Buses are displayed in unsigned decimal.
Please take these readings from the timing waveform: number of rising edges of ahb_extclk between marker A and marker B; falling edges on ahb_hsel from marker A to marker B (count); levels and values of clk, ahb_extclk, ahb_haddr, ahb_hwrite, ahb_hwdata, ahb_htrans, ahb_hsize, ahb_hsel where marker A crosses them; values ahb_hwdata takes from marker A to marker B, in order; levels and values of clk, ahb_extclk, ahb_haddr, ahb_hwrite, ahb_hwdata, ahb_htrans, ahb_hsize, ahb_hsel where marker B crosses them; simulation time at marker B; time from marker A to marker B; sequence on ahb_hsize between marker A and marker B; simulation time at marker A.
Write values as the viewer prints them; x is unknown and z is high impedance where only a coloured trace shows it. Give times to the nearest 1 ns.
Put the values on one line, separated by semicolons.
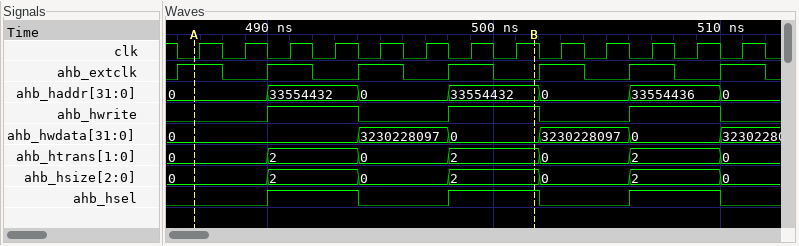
3; 1; clk=0, ahb_extclk=1, ahb_haddr=0, ahb_hwrite=0, ahb_hwdata=0, ahb_htrans=0, ahb_hsize=0, ahb_hsel=0; 0, 3230228097, 0; clk=1, ahb_extclk=0, ahb_haddr=33554432, ahb_hwrite=1, ahb_hwdata=0, ahb_htrans=2, ahb_hsize=2, ahb_hsel=1; 502 ns; 15 ns; 0, 2, 0, 2; 487 ns
